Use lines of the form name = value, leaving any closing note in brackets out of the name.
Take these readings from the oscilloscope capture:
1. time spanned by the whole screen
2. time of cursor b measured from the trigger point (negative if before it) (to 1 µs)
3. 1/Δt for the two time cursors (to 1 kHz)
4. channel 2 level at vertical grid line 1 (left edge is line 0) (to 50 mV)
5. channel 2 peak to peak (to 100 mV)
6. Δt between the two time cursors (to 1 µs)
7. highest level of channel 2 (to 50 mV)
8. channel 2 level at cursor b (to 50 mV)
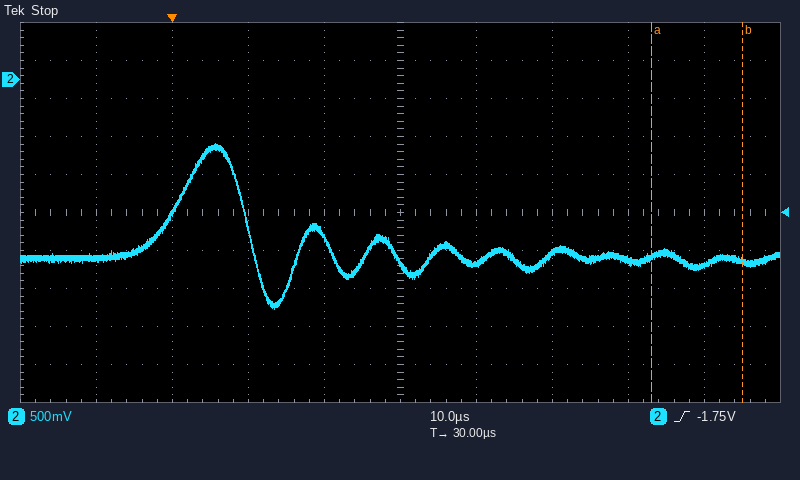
time spanned by the whole screen = 100 µs
time of cursor b measured from the trigger point (negative if before it) = +75 µs
1/Δt for the two time cursors = 83 kHz
channel 2 level at vertical grid line 1 (left edge is line 0) = -2.35 V
channel 2 peak to peak = 2.20 V
Δt between the two time cursors = 12 µs
highest level of channel 2 = -850 mV
channel 2 level at cursor b = -2.40 V
